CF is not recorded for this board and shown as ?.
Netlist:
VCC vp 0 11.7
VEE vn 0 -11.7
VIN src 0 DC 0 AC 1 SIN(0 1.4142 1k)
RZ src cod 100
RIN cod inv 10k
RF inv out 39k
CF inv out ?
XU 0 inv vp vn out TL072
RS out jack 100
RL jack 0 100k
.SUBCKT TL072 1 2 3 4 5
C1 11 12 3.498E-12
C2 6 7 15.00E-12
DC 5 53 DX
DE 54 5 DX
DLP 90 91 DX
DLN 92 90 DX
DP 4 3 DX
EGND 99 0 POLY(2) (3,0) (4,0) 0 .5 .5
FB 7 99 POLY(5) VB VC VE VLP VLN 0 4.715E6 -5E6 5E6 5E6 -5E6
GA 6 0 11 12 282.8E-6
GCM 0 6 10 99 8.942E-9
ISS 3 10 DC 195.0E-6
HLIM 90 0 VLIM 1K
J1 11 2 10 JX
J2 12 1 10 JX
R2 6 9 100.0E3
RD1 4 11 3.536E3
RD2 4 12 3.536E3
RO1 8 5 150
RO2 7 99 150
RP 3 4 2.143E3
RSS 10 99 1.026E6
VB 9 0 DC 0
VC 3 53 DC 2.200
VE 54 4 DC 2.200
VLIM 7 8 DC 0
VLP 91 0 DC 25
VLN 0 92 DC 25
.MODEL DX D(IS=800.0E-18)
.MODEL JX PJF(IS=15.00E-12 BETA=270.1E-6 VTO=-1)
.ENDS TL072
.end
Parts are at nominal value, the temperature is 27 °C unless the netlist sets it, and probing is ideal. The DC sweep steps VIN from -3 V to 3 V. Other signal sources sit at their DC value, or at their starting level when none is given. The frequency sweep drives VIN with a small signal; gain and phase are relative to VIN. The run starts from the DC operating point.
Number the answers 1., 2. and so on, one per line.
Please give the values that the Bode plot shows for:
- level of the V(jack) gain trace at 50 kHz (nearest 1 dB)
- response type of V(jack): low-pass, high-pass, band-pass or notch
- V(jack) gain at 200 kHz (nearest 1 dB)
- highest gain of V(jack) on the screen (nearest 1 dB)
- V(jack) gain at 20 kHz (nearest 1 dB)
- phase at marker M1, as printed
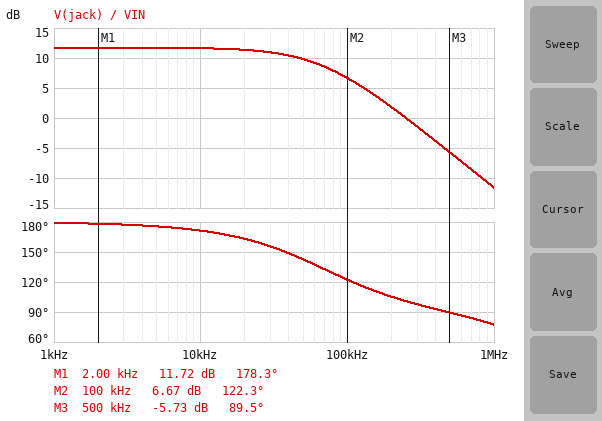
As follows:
1. 10 dB
2. low-pass
3. 2 dB
4. 12 dB
5. 11 dB
6. 178.3 deg
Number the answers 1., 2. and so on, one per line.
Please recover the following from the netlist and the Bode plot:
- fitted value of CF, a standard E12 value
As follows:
1. 56 pF
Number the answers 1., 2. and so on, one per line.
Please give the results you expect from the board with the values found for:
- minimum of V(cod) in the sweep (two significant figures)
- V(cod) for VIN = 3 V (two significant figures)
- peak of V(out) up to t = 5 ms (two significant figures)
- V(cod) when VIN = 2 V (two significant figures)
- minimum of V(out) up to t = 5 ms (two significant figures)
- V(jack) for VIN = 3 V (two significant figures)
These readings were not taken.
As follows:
1. -3.0 V
2. 3.0 V
3. 5.5 V
4. 2.0 V
5. -5.5 V
6. -10 V
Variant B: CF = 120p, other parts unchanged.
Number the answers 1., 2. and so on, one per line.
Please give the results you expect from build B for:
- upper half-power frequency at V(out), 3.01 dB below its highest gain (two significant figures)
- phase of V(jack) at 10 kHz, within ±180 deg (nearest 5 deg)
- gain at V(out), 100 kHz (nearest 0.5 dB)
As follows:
1. 33 kHz
2. 165 deg
3. 1.5 dB
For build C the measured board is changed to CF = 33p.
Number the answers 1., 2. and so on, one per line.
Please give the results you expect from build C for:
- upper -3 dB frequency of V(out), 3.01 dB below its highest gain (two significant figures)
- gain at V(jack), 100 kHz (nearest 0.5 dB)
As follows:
1. 110 kHz
2. 9.0 dB
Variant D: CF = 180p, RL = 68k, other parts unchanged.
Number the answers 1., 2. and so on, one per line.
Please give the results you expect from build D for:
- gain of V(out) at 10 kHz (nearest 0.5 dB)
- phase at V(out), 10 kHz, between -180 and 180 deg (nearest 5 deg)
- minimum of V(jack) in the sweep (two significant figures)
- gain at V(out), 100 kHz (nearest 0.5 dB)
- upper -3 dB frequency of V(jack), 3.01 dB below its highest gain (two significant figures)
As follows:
1. 11.0 dB
2. 155 deg
3. -10 V
4. -1.5 dB
5. 22 kHz
